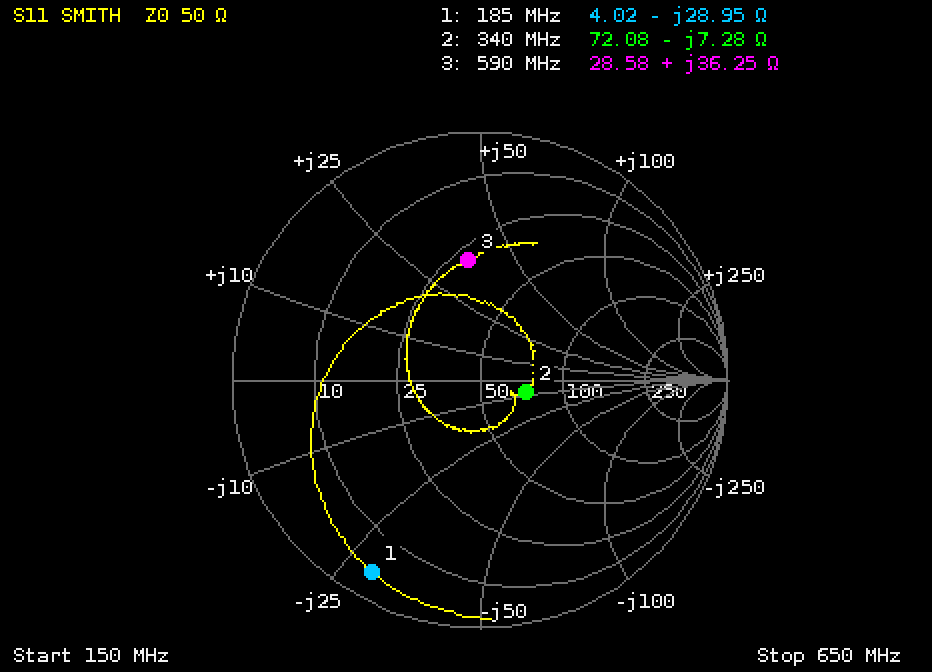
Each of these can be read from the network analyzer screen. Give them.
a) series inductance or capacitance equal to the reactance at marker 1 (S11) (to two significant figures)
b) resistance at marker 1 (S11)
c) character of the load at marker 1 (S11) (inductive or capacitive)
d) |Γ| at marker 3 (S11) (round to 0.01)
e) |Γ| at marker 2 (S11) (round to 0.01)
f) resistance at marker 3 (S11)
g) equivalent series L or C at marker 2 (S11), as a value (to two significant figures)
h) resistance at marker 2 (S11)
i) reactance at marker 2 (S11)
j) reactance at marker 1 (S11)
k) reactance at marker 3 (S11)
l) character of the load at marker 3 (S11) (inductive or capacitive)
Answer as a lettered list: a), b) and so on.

a) 30 pF
b) 4.02 Ω
c) capacitive
d) 0.49
e) 0.19
f) 28.58 Ω
g) 64 pF
h) 72.08 Ω
i) -7.28 Ω
j) -28.95 Ω
k) +36.25 Ω
l) inductive
